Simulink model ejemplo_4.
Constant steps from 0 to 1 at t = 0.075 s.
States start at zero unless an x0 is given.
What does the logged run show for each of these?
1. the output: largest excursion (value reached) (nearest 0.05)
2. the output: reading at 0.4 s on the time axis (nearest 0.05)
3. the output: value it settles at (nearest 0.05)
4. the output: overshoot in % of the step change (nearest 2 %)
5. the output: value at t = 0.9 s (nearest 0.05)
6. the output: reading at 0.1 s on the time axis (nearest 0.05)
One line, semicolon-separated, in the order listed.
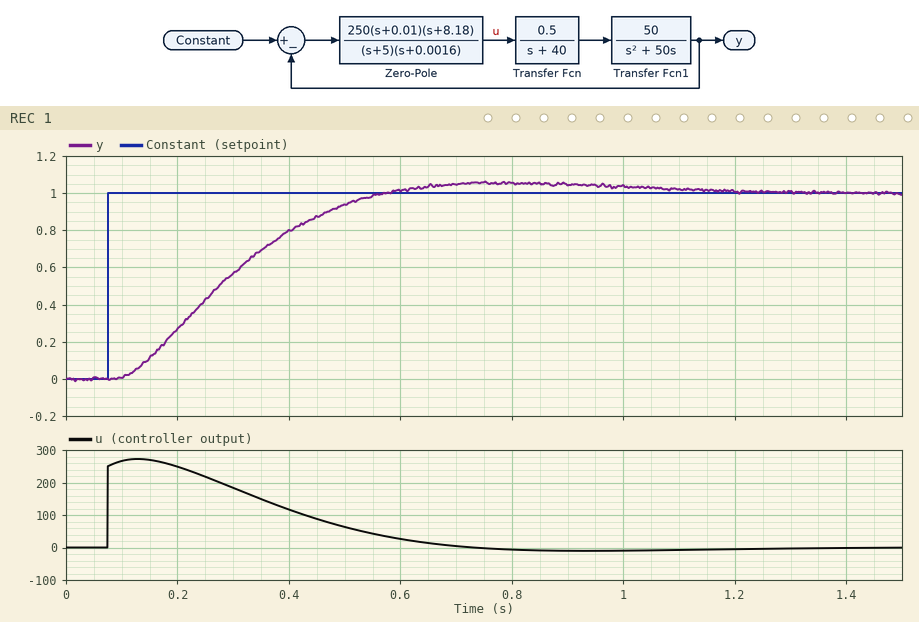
1.05; 0.80; 1.00; 6 %; 1.05; 0.00
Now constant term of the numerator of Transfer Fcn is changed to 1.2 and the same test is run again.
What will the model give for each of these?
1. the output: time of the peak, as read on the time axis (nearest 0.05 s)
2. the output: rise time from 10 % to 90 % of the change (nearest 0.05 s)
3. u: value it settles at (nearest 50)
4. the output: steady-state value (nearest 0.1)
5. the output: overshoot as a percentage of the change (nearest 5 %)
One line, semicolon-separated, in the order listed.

0.40 s; 0.15 s; 0; 1.0; 15 %
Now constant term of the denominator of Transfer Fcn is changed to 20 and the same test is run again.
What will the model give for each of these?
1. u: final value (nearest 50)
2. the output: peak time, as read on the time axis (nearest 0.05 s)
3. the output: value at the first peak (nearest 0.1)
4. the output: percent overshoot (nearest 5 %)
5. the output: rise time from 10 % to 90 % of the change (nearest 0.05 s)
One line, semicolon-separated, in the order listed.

0; 0.45 s; 1.2; 20 %; 0.15 s
